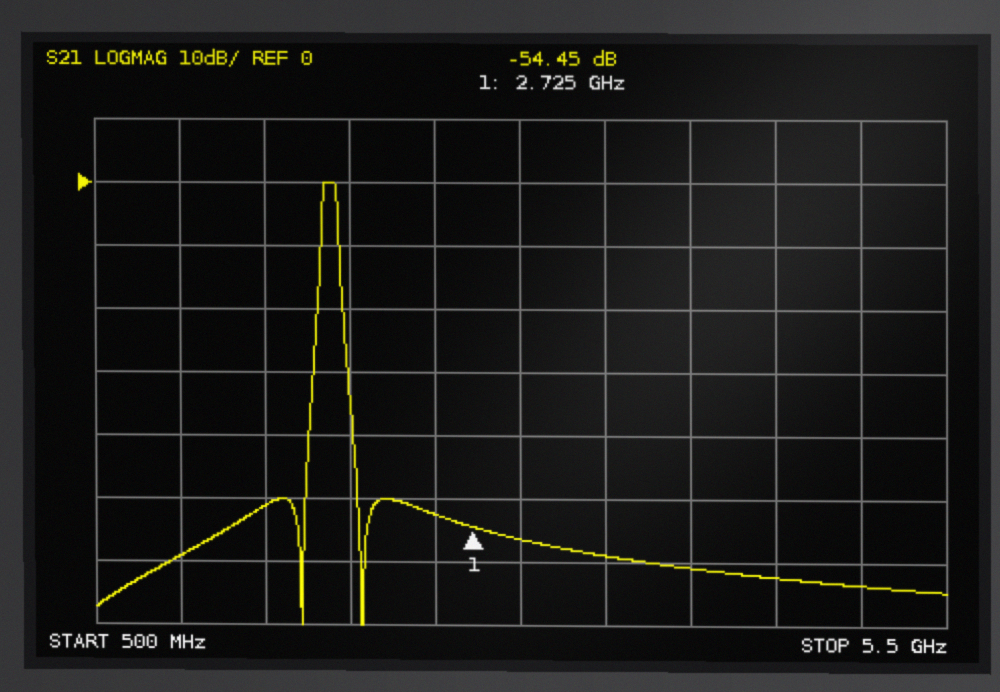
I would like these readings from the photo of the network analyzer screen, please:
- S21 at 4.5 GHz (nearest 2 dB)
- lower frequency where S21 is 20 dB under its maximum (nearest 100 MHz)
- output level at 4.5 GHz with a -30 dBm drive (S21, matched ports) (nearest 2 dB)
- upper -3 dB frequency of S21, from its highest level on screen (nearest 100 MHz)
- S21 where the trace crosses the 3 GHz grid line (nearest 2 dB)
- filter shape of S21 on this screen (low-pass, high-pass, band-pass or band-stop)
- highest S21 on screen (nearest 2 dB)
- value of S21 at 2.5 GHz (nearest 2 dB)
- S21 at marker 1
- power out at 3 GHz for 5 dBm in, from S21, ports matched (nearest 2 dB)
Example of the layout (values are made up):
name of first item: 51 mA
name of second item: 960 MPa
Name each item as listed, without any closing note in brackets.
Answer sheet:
S21 at 4.5 GHz: -62 dB
lower frequency where S21 is 20 dB under its maximum: 1.8 GHz
output level at 4.5 GHz with a -30 dBm drive (S21, matched ports): -92 dBm
upper -3 dB frequency of S21, from its highest level on screen: 1.9 GHz
S21 where the trace crosses the 3 GHz grid line: -56 dB
filter shape of S21 on this screen: band-pass
highest S21 on screen: 0 dB
value of S21 at 2.5 GHz: -52 dB
S21 at marker 1: -54.45 dB
power out at 3 GHz for 5 dBm in, from S21, ports matched: -52 dBm
